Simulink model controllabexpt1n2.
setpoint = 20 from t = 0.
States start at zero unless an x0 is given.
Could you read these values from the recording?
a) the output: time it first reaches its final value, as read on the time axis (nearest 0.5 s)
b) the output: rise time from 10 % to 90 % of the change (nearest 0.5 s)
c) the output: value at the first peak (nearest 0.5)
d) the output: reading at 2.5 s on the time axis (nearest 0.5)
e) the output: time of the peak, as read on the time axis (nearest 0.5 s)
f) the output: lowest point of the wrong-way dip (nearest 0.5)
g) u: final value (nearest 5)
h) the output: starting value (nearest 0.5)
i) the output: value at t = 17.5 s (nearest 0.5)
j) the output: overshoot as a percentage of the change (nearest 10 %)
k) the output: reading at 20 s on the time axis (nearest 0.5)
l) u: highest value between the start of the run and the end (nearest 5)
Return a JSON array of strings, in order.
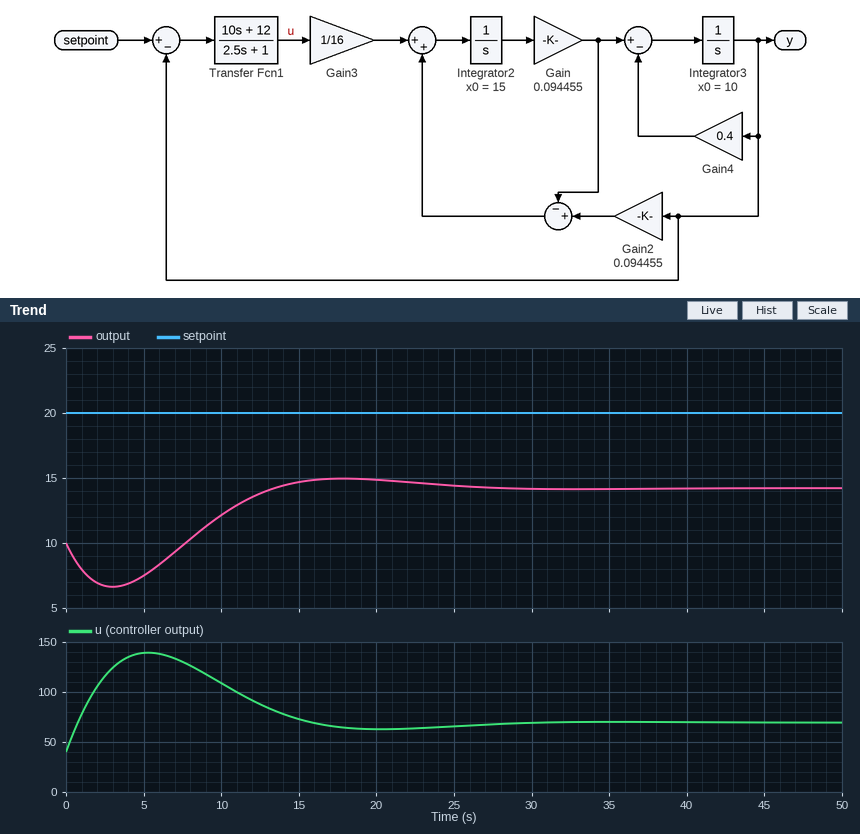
["13.5 s", "4.5 s", "15.0", "6.5", "18.0 s", "6.5", "70", "10.0", "15.0", "20 %", "15.0", "140"]
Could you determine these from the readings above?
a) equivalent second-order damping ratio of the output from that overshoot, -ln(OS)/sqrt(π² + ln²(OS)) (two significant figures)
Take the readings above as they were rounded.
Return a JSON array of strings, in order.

["0.46"]
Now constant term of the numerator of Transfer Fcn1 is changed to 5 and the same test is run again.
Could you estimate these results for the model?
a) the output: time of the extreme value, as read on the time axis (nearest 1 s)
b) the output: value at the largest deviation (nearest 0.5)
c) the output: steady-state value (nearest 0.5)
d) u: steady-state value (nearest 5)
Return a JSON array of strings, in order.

["4 s", "6.0", "10.0", "50"]
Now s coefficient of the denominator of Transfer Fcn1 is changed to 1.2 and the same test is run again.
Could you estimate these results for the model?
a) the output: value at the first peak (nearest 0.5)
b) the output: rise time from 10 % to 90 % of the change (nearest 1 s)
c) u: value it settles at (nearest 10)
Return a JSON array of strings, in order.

["14.5", "5 s", "70"]
